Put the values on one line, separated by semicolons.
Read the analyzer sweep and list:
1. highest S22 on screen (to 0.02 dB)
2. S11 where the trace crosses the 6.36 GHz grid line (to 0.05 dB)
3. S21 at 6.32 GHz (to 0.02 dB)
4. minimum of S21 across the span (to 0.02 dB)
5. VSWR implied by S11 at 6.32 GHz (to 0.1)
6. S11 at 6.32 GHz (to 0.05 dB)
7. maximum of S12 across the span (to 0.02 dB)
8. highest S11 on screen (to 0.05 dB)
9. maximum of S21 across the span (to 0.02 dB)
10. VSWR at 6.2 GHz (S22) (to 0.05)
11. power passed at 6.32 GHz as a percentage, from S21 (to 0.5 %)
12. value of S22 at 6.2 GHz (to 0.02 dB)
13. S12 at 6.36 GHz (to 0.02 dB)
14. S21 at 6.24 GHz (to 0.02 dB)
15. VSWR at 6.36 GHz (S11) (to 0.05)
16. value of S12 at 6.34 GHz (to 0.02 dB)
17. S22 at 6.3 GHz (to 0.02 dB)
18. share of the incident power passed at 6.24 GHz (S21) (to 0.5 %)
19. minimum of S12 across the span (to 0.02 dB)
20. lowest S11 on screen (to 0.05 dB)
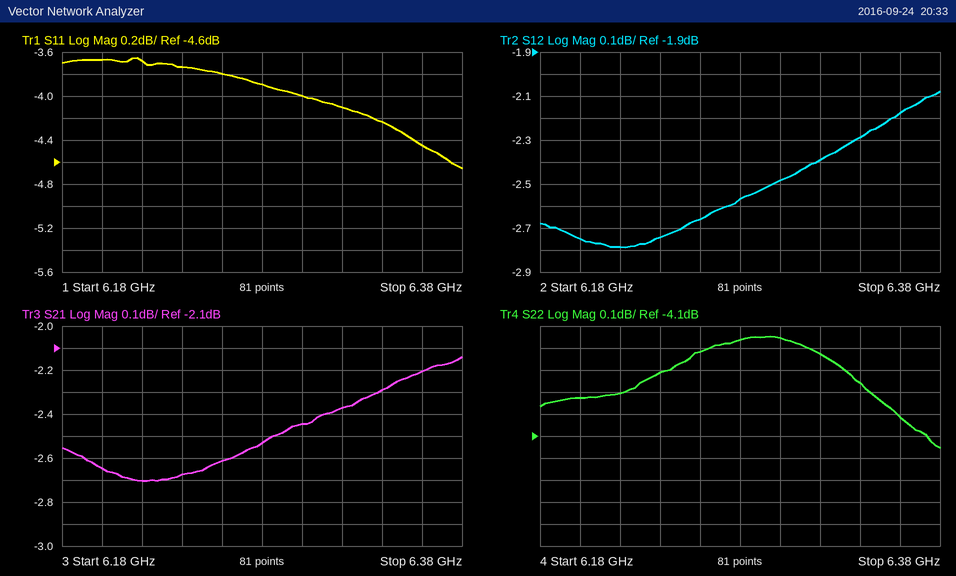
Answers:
-3.64 dB; -4.45 dB; -2.38 dB; -2.70 dB; 4.3; -4.10 dB; -2.08 dB; -3.65 dB; -2.14 dB; 4.50; 58.0 %; -3.92 dB; -2.18 dB; -2.68 dB; 4.00; -2.28 dB; -3.66 dB; 54.0 %; -2.78 dB; -4.65 dB
